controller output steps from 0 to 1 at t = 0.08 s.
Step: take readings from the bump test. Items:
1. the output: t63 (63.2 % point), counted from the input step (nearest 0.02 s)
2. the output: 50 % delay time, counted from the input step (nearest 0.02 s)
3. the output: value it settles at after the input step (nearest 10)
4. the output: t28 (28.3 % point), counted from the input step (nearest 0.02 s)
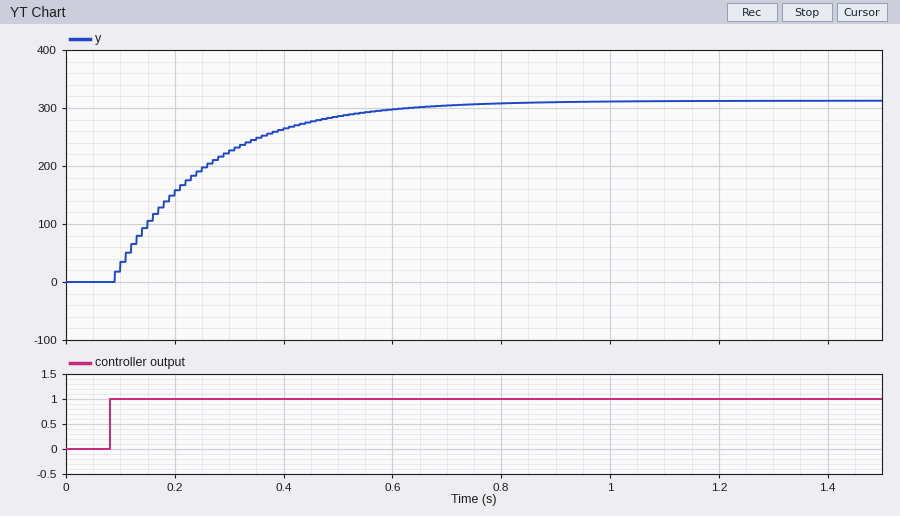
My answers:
0.18 s
0.12 s
310
0.06 s
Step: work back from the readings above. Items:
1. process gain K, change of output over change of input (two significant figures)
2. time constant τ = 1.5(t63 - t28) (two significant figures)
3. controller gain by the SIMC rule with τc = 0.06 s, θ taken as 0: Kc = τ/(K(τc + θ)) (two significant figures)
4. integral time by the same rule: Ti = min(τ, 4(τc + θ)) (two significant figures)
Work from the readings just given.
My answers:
310
0.18 s
0.0097
0.18 s
